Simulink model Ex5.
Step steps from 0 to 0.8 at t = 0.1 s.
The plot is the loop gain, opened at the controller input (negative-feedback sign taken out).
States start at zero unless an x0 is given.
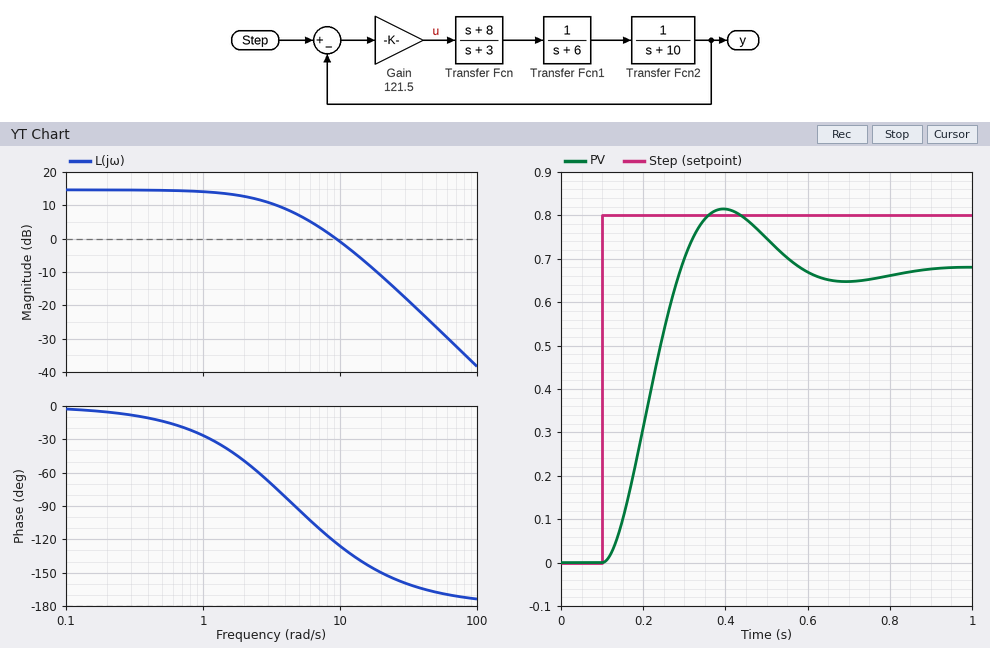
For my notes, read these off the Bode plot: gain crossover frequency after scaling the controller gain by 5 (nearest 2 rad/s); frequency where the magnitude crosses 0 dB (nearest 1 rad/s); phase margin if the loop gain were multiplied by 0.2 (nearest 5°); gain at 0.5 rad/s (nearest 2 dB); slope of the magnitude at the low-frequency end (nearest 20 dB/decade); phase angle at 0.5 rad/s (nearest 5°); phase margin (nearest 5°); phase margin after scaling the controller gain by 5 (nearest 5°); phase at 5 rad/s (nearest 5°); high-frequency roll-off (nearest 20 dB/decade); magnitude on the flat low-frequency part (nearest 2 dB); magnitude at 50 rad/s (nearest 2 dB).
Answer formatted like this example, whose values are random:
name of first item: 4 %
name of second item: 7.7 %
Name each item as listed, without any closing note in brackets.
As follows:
gain crossover frequency after scaling the controller gain by 5: 24 rad/s
frequency where the magnitude crosses 0 dB: 9 rad/s
phase margin if the loop gain were multiplied by 0.2: 150°
gain at 0.5 rad/s: 14 dB
slope of the magnitude at the low-frequency end: 0 dB/decade
phase angle at 0.5 rad/s: -15°
phase margin: 55°
phase margin after scaling the controller gain by 5: 25°
phase at 5 rad/s: -95°
high-frequency roll-off: -40 dB/decade
magnitude on the flat low-frequency part: 14 dB
magnitude at 50 rad/s: -26 dB
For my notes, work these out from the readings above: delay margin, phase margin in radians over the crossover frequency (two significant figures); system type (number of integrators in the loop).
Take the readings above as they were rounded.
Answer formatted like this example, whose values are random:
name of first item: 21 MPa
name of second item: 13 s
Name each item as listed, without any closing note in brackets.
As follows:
delay margin, phase margin in radians over the crossover frequency: 0.11 s
system type: 0
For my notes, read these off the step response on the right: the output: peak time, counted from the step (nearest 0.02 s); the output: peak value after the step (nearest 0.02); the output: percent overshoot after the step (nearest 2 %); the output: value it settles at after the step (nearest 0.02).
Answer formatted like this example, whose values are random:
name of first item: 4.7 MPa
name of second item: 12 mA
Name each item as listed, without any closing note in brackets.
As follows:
the output: peak time, counted from the step: 0.30 s
the output: peak value after the step: 0.82
the output: percent overshoot after the step: 20 %
the output: value it settles at after the step: 0.68
